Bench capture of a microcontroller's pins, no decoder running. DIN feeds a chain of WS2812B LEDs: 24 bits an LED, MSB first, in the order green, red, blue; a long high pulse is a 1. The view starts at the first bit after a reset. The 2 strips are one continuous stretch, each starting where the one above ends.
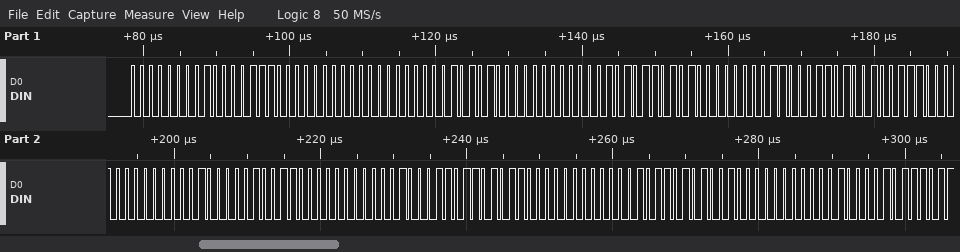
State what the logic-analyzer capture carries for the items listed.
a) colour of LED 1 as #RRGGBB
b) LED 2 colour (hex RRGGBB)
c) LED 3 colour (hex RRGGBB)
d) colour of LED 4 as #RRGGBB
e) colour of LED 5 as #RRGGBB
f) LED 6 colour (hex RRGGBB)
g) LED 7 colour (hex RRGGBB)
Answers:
#870000
#150000
#D40A03
#4E1A00
#260800
#6B2300
#520B00
